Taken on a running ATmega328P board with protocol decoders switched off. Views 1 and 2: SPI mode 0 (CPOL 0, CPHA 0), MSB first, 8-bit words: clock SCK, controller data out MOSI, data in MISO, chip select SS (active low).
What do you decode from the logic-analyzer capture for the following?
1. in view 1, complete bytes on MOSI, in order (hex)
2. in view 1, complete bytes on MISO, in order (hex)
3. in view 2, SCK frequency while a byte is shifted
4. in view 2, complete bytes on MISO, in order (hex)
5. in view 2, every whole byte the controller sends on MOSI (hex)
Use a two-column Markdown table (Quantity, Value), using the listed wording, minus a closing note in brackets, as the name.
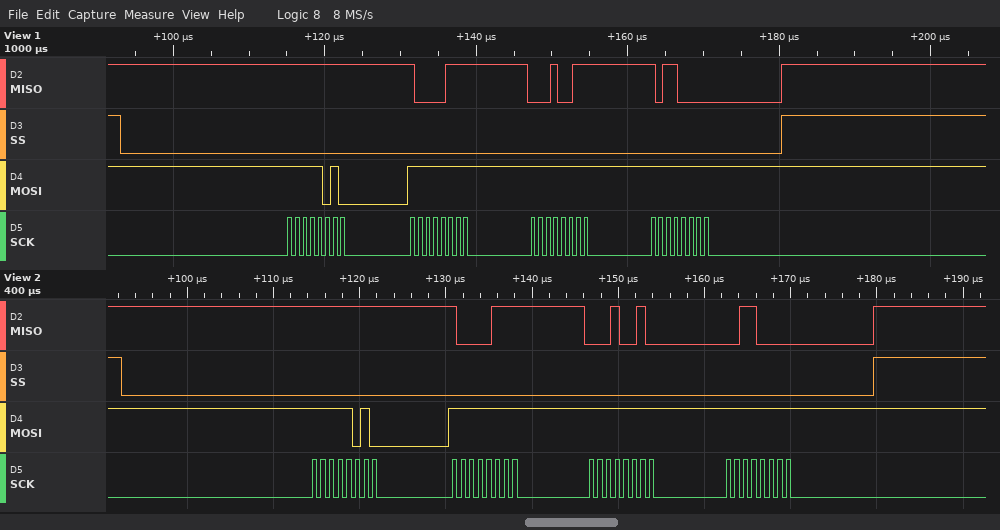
| Quantity | Value |
|---|---|
| in view 1, complete bytes on MOSI, in order | FA FF FF FF |
| in view 1, complete bytes on MISO, in order | FF 87 13 B0 |
| in view 2, SCK frequency while a byte is shifted | 1 MHz |
| in view 2, complete bytes on MISO, in order | FF 87 12 30 |
| in view 2, every whole byte the controller sends on MOSI | FA FF FF FF |
